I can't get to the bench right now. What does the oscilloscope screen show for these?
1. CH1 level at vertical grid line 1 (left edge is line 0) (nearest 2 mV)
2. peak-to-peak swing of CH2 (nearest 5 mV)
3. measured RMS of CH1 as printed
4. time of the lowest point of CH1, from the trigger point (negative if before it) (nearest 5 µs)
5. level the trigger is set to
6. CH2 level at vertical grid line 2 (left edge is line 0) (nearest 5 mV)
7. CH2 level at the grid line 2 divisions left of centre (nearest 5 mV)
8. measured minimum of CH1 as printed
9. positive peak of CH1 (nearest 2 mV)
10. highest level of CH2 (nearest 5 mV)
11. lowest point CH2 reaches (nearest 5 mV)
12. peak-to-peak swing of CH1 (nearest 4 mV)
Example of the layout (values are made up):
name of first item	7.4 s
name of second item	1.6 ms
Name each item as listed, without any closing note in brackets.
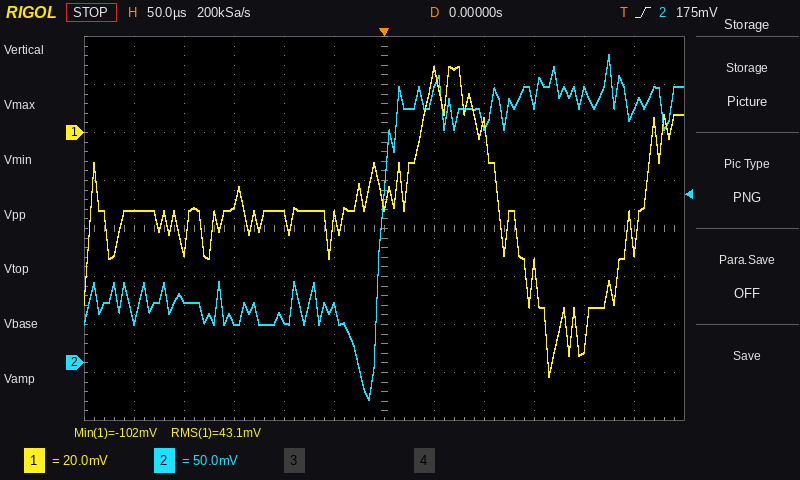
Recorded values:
CH1 level at vertical grid line 1 (left edge is line 0)	-32 mV
peak-to-peak swing of CH2	360 mV
measured RMS of CH1 as printed	43.1 mV
time of the lowest point of CH1, from the trigger point (negative if before it)	+165 µs
level the trigger is set to	175 mV
CH2 level at vertical grid line 2 (left edge is line 0)	65 mV
CH2 level at the grid line 2 divisions left of centre	45 mV
measured minimum of CH1 as printed	-102 mV
positive peak of CH1	28 mV
highest level of CH2	320 mV
lowest point CH2 reaches	-40 mV
peak-to-peak swing of CH1	128 mV
